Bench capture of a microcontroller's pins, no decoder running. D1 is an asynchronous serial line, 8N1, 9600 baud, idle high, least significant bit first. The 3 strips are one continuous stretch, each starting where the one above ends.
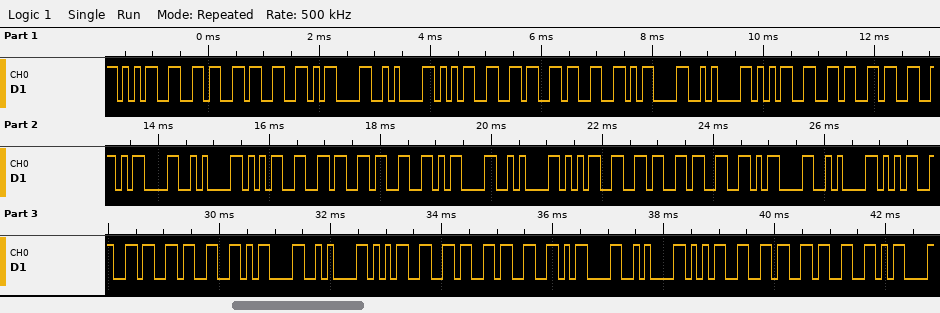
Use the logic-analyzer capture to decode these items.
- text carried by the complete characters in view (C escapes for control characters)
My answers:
"563\r\n563\r\n563\r\n563\r\n563\r\n563\r\n563\r\n563\r"
